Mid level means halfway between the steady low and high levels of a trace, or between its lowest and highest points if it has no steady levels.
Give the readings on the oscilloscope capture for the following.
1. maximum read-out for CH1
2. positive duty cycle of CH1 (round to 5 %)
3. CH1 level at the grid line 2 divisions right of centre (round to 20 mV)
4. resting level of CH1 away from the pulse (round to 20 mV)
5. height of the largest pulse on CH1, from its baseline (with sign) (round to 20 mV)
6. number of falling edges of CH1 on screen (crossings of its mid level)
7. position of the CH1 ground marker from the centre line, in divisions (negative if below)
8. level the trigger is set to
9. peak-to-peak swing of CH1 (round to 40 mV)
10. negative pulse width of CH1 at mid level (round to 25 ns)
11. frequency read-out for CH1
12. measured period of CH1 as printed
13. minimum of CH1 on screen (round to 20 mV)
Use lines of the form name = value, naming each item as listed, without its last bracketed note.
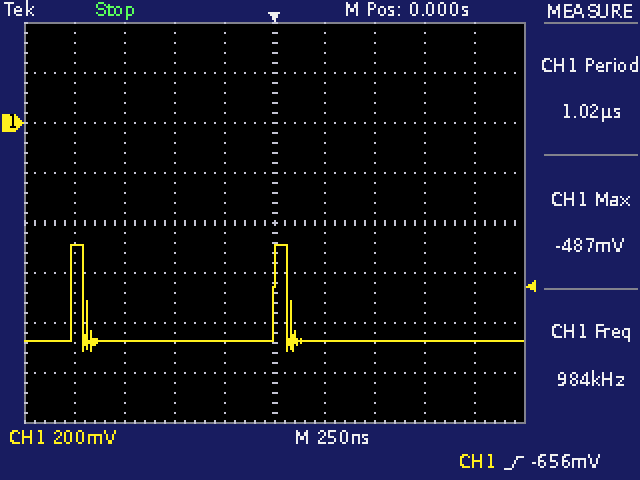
maximum read-out for CH1 = -487 mV
positive duty cycle of CH1 = 5 %
CH1 level at the grid line 2 divisions right of centre = -880 mV
resting level of CH1 away from the pulse = -880 mV
height of the largest pulse on CH1, from its baseline (with sign) = +380 mV
number of falling edges of CH1 on screen = 2
position of the CH1 ground marker from the centre line, in divisions = +2.0 div
level the trigger is set to = -656 mV
peak-to-peak swing of CH1 = 440 mV
negative pulse width of CH1 at mid level = 950 ns
frequency read-out for CH1 = 984 kHz
measured period of CH1 as printed = 1.02 µs
minimum of CH1 on screen = -920 mV
